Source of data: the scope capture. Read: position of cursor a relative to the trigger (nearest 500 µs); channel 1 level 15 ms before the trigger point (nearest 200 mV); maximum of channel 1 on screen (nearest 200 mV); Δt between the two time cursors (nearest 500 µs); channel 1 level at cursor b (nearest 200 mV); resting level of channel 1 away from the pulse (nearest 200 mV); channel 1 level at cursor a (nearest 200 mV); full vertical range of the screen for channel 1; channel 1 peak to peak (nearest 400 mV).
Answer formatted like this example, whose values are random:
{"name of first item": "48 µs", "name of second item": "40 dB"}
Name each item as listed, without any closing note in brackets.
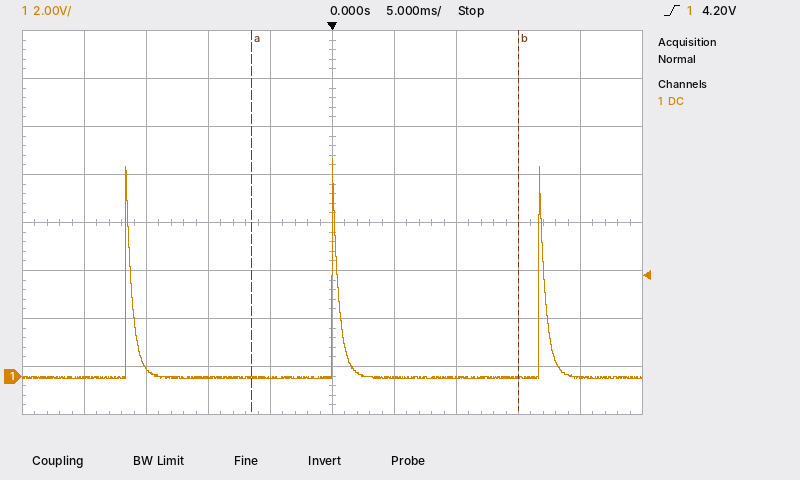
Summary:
{"position of cursor a relative to the trigger": "-6.5 ms", "channel 1 level 15 ms before the trigger point": "400 mV", "maximum of channel 1 on screen": "9.0 V", "Δt between the two time cursors": "21.5 ms", "channel 1 level at cursor b": "0.0 V", "resting level of channel 1 away from the pulse": "0.0 V", "channel 1 level at cursor a": "0.0 V", "full vertical range of the screen for channel 1": "16 V", "channel 1 peak to peak": "9.2 V"}
